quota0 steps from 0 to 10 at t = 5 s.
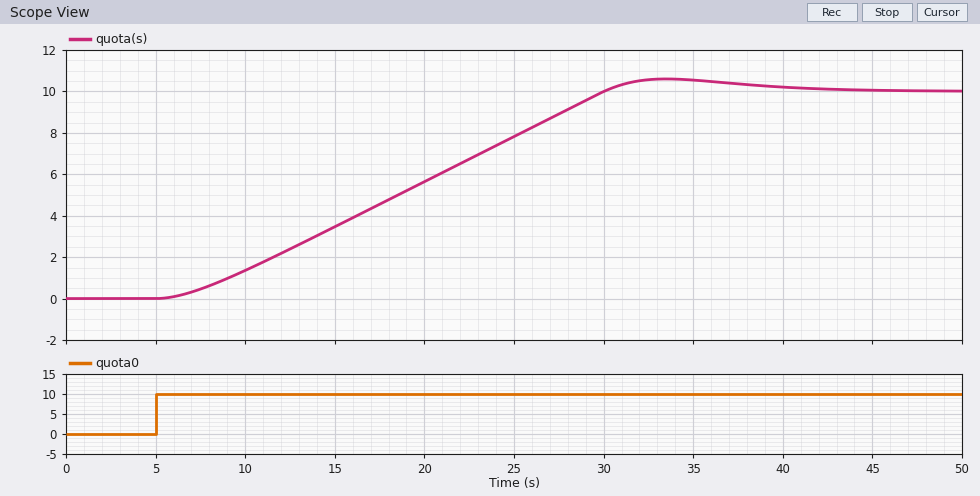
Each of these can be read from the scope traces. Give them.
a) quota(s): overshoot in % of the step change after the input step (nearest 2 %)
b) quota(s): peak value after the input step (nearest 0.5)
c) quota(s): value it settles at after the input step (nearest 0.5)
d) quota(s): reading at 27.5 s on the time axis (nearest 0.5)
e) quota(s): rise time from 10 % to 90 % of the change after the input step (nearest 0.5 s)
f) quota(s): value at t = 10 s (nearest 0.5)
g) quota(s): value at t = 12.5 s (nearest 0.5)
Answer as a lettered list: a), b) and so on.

a) 6 %
b) 10.5
c) 10.0
d) 9.0
e) 18.5 s
f) 1.5
g) 2.5
